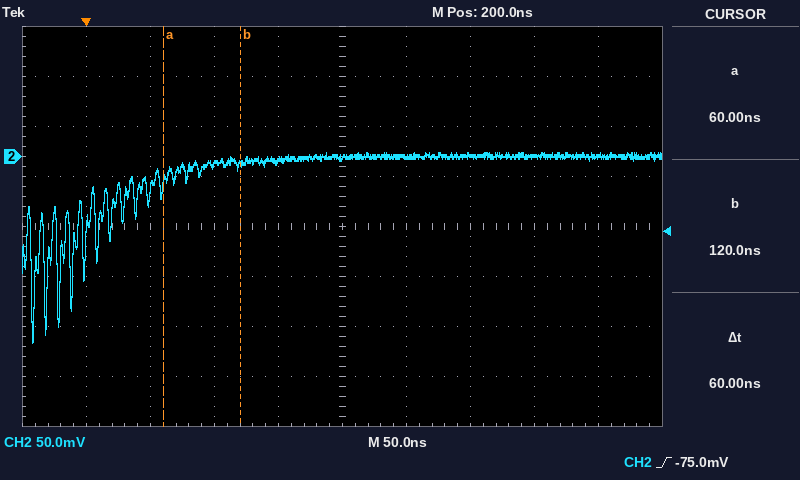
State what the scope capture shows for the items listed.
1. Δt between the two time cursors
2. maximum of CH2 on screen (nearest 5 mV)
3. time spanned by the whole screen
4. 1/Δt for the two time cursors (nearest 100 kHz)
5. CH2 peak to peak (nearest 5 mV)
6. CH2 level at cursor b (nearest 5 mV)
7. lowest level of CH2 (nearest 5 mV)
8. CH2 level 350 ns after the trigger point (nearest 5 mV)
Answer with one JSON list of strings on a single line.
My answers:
["60 ns", "5 mV", "500 ns", "16.7 MHz", "190 mV", "-10 mV", "-185 mV", "0 mV"]
